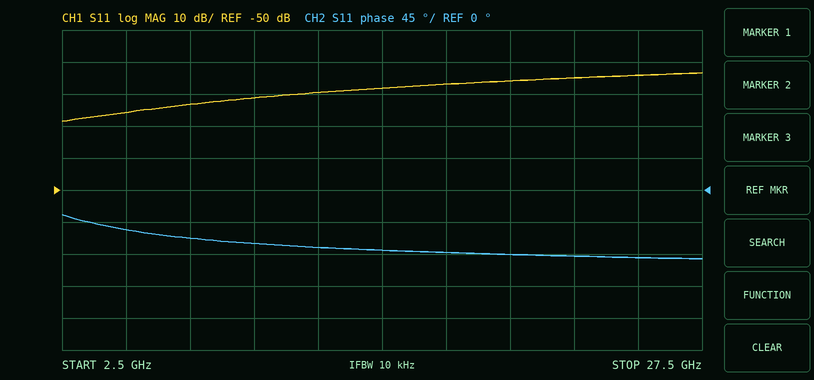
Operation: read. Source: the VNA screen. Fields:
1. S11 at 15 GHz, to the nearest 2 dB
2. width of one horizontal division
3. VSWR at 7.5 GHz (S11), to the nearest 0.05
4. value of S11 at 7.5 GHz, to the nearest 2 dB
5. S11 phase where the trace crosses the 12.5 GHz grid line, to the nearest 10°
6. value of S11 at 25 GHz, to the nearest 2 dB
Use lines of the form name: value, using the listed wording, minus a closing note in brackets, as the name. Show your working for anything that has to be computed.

S11 at 15 GHz, to the nearest 2 dB: -18 dB
width of one horizontal division: 2.5 GHz
VSWR at 7.5 GHz (S11), to the nearest 0.05: |Γ| = 10^(-24/20) = 0.0631; VSWR = (1 + 0.0631)/(1 − 0.0631) ≈ 1.13, so 1.15 to the nearest 0.05
value of S11 at 7.5 GHz, to the nearest 2 dB: -24 dB
S11 phase where the trace crosses the 12.5 GHz grid line, to the nearest 10°: -80°
value of S11 at 25 GHz, to the nearest 2 dB: -14 dB
